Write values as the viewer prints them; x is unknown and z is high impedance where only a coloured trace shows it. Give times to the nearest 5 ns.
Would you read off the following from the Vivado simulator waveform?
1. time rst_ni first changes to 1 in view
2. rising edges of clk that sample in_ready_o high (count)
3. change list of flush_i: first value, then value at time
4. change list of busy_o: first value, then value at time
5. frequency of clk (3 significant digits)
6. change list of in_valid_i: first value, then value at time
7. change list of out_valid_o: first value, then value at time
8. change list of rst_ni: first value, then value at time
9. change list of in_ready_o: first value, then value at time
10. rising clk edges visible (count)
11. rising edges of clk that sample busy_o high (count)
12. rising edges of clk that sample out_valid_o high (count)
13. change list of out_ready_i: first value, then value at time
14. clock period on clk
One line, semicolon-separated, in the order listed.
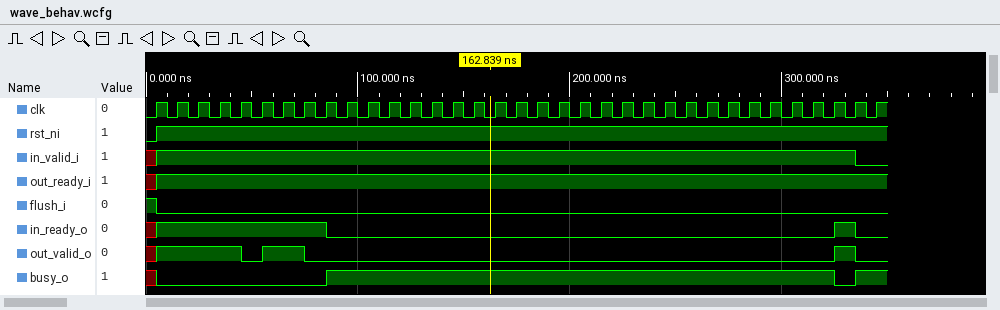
5 ns; 9; 1, 0 at 5 ns; x, 0 at 5 ns, 1 at 85 ns, 0 at 325 ns, 1 at 335 ns; 100 MHz; x, 1 at 5 ns, 0 at 335 ns; x, 1 at 5 ns, 0 at 45 ns, 1 at 55 ns, 0 at 75 ns, 1 at 325 ns, 0 at 335 ns; 0, 1 at 5 ns; x, 1 at 5 ns, 0 at 85 ns, 1 at 325 ns, 0 at 335 ns; 35; 25; 7; x, 1 at 5 ns; 10 ns
